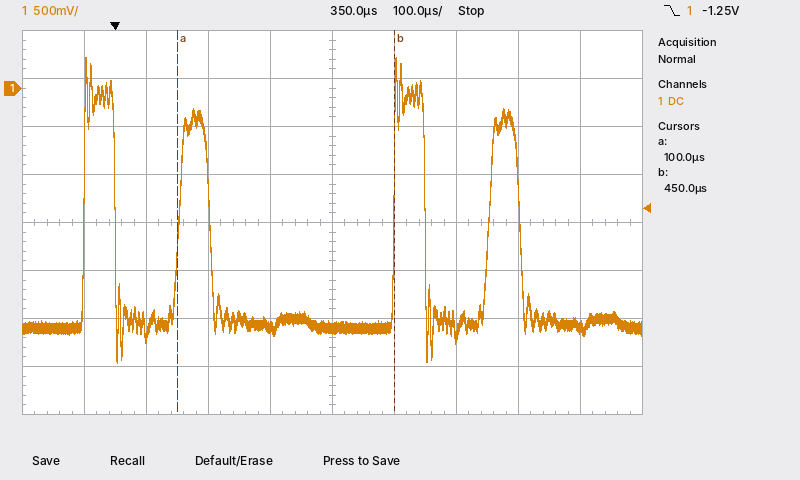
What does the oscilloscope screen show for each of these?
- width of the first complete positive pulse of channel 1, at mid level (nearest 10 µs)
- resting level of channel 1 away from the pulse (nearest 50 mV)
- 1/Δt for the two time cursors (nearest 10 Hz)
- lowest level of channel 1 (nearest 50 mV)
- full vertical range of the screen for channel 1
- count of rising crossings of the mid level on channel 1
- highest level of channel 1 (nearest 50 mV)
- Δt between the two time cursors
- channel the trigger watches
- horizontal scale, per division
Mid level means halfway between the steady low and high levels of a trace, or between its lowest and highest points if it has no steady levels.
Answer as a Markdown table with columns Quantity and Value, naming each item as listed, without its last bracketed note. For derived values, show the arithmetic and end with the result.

| Quantity | Value |
|---|---|
| width of the first complete positive pulse of channel 1, at mid level | 50 µs |
| resting level of channel 1 away from the pulse | -2.45 V |
| 1/Δt for the two time cursors | 1 / 350 µs ≈ 2.86 kHz |
| lowest level of channel 1 | -2.85 V |
| full vertical range of the screen for channel 1 | 4 V |
| count of rising crossings of the mid level on channel 1 | 4 |
| highest level of channel 1 | 300 mV |
| Δt between the two time cursors | 450 µs − (100 µs) = 350 µs |
| channel the trigger watches | channel 1 |
| horizontal scale, per division | 100 µs |
